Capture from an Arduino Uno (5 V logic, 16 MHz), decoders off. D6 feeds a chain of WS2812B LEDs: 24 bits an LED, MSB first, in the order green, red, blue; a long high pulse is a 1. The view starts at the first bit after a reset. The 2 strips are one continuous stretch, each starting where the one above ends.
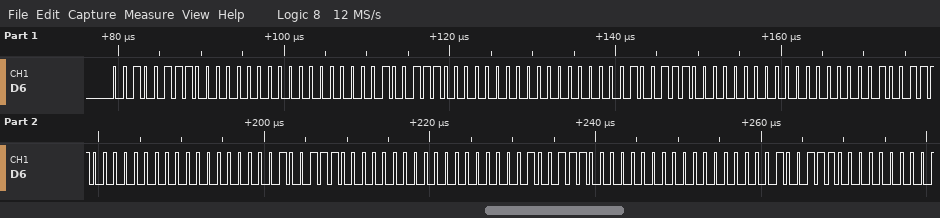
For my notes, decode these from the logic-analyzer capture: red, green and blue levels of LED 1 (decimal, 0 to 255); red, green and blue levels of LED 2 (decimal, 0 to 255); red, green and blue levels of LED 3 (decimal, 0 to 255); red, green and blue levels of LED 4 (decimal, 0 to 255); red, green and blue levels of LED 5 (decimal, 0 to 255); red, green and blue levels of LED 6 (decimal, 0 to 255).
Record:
0, 39, 0
0, 39, 0
0, 39, 0
0, 39, 0
0, 39, 0
0, 39, 0
